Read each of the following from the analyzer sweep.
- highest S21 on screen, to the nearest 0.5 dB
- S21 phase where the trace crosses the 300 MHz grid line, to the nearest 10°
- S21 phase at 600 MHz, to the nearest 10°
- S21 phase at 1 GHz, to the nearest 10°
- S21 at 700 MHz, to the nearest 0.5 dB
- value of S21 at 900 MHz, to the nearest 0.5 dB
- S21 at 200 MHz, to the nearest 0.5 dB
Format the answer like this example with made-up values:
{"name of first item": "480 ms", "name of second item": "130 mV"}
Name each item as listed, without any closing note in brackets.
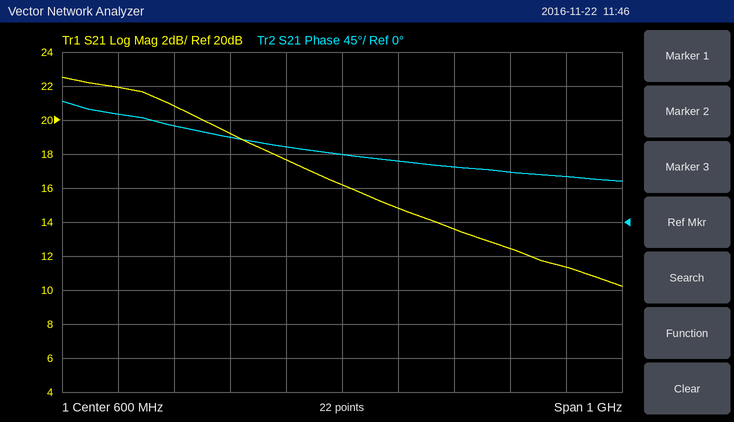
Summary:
{"highest S21 on screen, to the nearest 0.5 dB": "22.5 dB", "S21 phase where the trace crosses the 300 MHz grid line, to the nearest 10°": "130°", "S21 phase at 600 MHz, to the nearest 10°": "90°", "S21 phase at 1 GHz, to the nearest 10°": "60°", "S21 at 700 MHz, to the nearest 0.5 dB": "15.0 dB", "value of S21 at 900 MHz, to the nearest 0.5 dB": "12.5 dB", "S21 at 200 MHz, to the nearest 0.5 dB": "22.0 dB"}
